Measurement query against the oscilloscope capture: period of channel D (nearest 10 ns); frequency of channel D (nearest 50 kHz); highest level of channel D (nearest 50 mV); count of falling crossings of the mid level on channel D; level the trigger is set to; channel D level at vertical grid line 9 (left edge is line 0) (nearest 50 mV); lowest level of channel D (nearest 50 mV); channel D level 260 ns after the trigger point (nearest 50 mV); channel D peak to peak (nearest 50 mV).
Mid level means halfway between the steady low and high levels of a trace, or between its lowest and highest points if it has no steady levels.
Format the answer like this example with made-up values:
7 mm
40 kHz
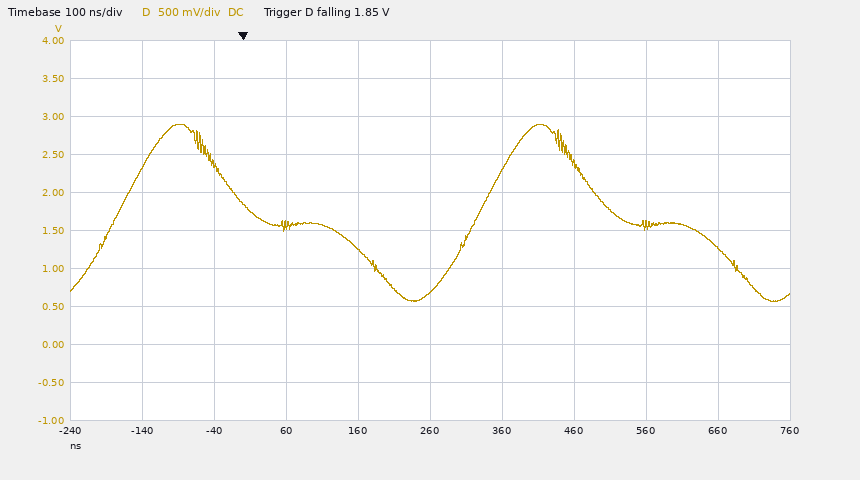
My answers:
500 ns
2.00 MHz
2.90 V
2
1.85 V
1.25 V
550 mV
700 mV
2.35 V
